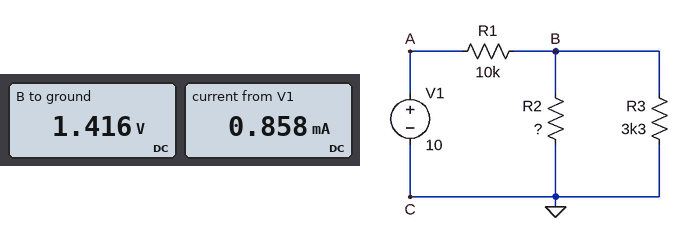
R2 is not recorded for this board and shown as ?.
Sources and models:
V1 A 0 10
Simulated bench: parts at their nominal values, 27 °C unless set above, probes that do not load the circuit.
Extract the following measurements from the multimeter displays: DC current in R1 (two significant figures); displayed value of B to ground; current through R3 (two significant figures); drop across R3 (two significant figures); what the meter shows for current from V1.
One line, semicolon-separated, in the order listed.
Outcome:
860 µA; 1.416 V; 430 µA; 1.4 V; 0.858 mA
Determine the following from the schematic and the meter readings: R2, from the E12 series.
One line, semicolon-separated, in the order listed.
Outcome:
3.3 kΩ
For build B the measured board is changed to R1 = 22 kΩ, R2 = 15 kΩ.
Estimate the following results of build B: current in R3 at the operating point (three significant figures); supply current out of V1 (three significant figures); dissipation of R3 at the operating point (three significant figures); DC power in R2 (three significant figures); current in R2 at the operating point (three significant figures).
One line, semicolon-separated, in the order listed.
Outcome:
332 µA; 405 µA; 363 µW; 79.9 µW; 73.0 µA
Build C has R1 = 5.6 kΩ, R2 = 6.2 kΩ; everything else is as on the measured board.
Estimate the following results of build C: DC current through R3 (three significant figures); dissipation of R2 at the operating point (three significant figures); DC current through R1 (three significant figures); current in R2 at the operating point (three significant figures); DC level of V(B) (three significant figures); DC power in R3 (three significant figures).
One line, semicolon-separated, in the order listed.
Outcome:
842 µA; 1.24 mW; 1.29 mA; 448 µA; 2.78 V; 2.34 mW
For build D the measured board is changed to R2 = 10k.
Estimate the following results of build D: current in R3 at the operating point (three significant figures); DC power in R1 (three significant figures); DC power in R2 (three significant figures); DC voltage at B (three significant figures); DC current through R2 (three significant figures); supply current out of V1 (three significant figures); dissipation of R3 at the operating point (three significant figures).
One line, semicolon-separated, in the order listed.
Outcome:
602 µA; 6.42 mW; 395 µW; 1.99 V; 199 µA; 801 µA; 1.20 mW
